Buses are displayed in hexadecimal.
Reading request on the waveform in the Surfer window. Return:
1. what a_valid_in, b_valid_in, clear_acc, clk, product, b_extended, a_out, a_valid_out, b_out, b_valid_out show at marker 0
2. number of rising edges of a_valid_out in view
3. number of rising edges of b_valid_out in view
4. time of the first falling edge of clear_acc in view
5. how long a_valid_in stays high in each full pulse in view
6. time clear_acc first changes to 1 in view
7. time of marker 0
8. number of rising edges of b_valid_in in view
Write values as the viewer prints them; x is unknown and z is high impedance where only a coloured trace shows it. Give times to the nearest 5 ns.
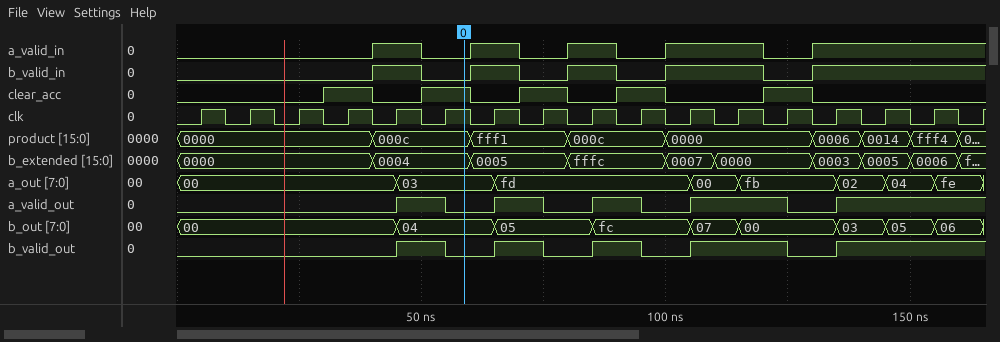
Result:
a_valid_in=0, b_valid_in=0, clear_acc=1, clk=1, product=000c, b_extended=0004, a_out=03, a_valid_out=0, b_out=04, b_valid_out=0
5
5
40 ns
10 ns, 10 ns, 10 ns, 20 ns
30 ns
60 ns
5
